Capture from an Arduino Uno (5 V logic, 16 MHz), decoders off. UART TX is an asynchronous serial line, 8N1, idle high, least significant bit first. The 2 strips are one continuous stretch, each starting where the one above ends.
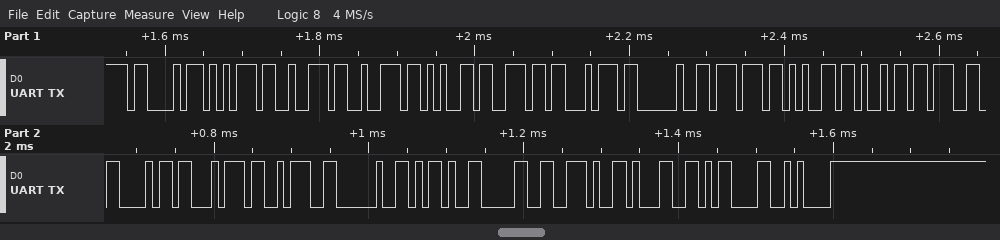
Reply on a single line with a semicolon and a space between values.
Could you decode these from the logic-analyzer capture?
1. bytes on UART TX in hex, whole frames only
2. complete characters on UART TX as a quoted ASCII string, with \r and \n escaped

43 75 72 72 65 6E 74 20 77 65 69 67 68 74 3A 20 2D 30 2E 31 0D 0A; "Current weight: -0.1\r\n"
